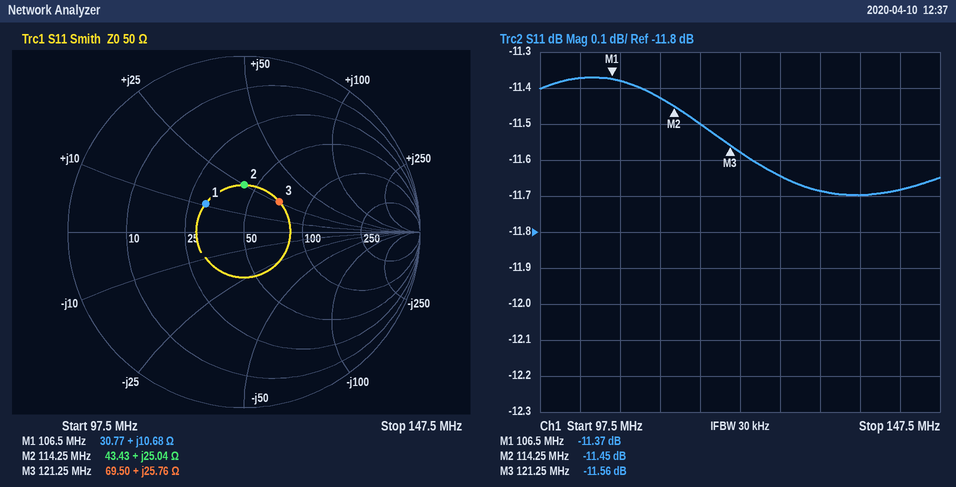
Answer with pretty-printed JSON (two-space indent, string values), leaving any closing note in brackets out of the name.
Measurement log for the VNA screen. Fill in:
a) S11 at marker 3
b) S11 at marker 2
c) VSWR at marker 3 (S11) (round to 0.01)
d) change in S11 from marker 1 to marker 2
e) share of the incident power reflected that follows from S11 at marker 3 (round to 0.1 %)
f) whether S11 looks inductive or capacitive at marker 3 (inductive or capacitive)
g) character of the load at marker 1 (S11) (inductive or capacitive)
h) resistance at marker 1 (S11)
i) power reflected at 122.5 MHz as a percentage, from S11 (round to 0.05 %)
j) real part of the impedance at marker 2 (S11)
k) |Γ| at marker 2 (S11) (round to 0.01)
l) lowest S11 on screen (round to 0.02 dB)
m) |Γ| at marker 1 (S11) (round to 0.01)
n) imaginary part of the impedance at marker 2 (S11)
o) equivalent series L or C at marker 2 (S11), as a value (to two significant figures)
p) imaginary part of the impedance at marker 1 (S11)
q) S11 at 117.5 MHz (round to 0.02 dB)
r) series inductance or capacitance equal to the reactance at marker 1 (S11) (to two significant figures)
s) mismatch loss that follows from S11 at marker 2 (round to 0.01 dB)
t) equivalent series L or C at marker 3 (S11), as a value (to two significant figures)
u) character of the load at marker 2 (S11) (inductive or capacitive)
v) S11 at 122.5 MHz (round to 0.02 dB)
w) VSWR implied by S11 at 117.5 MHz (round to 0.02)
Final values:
{
  "S11 at marker 3": "-11.56 dB",
  "S11 at marker 2": "-11.45 dB",
  "VSWR at marker 3 (S11)": "1.72",
  "change in S11 from marker 1 to marker 2": "-0.08 dB",
  "share of the incident power reflected that follows from S11 at marker 3": "7.0 %",
  "whether S11 looks inductive or capacitive at marker 3": "inductive",
  "character of the load at marker 1 (S11)": "inductive",
  "resistance at marker 1": "30.77 Ω",
  "power reflected at 122.5 MHz as a percentage, from S11": "6.95 %",
  "real part of the impedance at marker 2": "43.43 Ω",
  "|Γ| at marker 2 (S11)": "0.27",
  "lowest S11 on screen": "-11.70 dB",
  "|Γ| at marker 1 (S11)": "0.27",
  "imaginary part of the impedance at marker 2": "+25.04 Ω",
  "equivalent series L or C at marker 2 (S11), as a value": "35 nH",
  "imaginary part of the impedance at marker 1": "+10.68 Ω",
  "S11 at 117.5 MHz": "-11.50 dB",
  "series inductance or capacitance equal to the reactance at marker 1 (S11)": "16 nH",
  "mismatch loss that follows from S11 at marker 2": "0.32 dB",
  "equivalent series L or C at marker 3 (S11), as a value": "34 nH",
  "character of the load at marker 2 (S11)": "inductive",
  "S11 at 122.5 MHz": "-11.58 dB",
  "VSWR implied by S11 at 117.5 MHz": "1.72"
}
